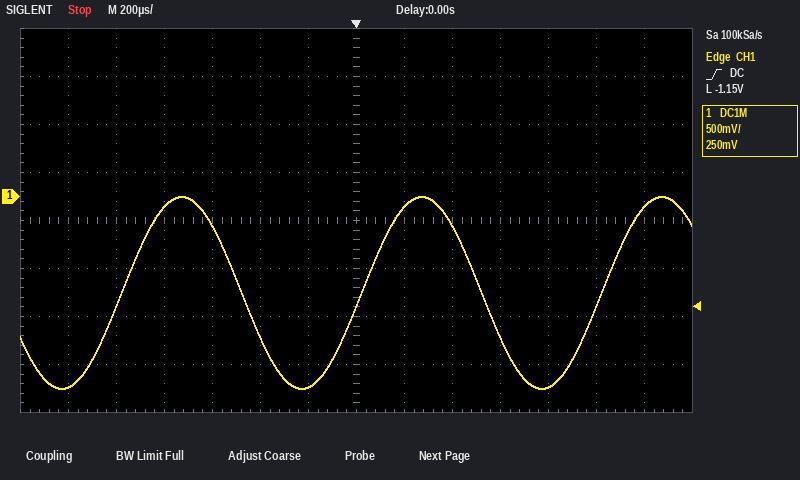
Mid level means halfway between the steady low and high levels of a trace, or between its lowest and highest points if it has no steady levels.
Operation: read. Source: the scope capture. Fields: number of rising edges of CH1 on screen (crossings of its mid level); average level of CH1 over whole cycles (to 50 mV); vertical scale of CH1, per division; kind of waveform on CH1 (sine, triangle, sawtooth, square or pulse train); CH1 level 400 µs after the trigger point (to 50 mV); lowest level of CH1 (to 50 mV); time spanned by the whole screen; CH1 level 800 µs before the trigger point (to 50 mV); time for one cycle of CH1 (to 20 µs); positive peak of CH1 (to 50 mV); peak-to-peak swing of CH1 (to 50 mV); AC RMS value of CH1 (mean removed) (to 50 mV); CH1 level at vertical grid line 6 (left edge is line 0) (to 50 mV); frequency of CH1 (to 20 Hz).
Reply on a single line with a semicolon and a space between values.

3; -1.00 V; 500 mV; sine; -300 mV; -2.00 V; 2.8 ms; -100 mV; 1.00 ms; 0 mV; 2.00 V; 700 mV; -2.00 V; 1.00 kHz
